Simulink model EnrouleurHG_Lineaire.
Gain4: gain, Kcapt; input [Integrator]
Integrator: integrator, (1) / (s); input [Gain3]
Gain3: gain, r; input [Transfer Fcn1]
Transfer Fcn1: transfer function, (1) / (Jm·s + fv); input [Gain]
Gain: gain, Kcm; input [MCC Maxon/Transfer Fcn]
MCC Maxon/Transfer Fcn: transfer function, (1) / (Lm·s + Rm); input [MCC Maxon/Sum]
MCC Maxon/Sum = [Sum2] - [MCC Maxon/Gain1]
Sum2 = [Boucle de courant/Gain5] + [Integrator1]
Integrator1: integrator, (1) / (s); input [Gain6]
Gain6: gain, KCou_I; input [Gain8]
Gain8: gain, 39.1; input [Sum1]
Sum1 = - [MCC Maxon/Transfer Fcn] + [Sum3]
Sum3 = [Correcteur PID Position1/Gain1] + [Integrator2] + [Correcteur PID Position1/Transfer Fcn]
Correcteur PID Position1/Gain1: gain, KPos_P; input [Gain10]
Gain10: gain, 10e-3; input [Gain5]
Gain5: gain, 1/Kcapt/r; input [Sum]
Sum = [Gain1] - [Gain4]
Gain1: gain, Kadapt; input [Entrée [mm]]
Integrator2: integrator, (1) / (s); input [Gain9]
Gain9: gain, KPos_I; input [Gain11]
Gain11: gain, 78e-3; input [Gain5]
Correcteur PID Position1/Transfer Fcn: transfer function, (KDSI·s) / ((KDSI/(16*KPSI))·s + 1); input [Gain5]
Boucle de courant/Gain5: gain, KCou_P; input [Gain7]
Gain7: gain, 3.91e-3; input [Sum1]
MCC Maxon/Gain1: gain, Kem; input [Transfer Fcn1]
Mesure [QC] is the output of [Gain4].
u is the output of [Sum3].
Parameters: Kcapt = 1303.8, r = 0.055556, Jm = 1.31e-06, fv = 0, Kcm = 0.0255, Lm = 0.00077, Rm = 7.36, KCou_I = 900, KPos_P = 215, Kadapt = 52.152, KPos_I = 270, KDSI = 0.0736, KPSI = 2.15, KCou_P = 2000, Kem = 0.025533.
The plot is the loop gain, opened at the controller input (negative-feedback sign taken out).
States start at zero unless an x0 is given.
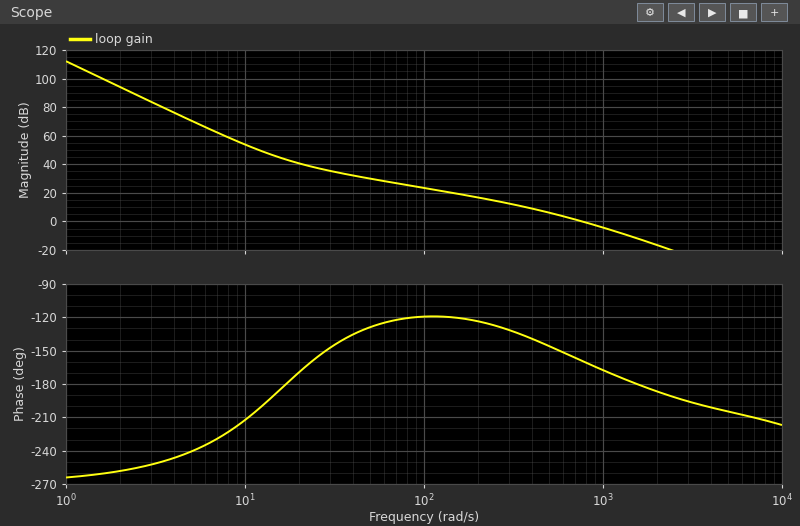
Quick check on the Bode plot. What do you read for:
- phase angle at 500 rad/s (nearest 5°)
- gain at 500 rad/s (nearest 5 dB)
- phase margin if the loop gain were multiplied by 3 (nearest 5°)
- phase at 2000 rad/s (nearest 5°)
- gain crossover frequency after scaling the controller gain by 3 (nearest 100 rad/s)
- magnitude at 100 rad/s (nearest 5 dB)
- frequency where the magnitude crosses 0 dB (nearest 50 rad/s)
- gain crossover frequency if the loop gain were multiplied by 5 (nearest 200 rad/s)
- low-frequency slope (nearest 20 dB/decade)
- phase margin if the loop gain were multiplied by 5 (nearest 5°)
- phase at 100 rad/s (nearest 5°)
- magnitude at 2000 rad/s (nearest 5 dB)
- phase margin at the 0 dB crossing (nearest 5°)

-145°
5 dB
5°
-185°
1400 rad/s
25 dB
750 rad/s
1800 rad/s
-60 dB/decade
-5°
-120°
-15 dB
20°
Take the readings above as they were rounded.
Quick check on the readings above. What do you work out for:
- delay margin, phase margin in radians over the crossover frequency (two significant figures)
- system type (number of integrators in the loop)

0.00047 s
3
